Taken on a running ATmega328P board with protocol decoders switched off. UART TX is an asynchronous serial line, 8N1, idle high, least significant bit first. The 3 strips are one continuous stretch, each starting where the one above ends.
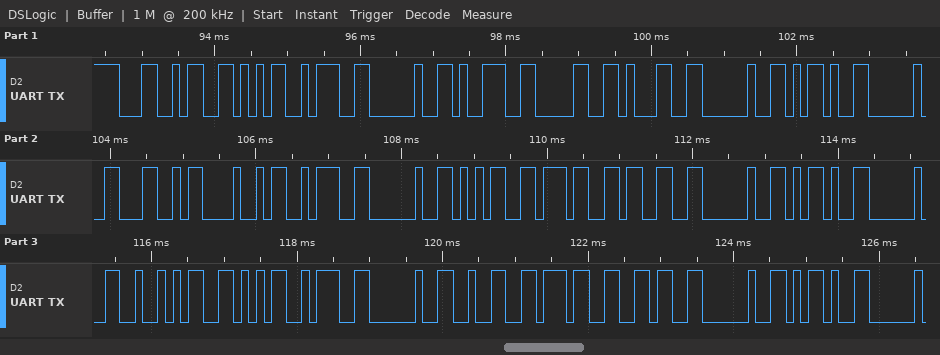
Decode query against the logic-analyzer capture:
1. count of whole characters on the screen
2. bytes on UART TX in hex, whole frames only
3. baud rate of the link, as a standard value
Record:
29
4C 56 3A 20 39 30 31 20 2D 20 4C 48 3A 20 35 37 33 20 2D 20 52 56 3A 20 32 37 36 20 2D
9600 baud
